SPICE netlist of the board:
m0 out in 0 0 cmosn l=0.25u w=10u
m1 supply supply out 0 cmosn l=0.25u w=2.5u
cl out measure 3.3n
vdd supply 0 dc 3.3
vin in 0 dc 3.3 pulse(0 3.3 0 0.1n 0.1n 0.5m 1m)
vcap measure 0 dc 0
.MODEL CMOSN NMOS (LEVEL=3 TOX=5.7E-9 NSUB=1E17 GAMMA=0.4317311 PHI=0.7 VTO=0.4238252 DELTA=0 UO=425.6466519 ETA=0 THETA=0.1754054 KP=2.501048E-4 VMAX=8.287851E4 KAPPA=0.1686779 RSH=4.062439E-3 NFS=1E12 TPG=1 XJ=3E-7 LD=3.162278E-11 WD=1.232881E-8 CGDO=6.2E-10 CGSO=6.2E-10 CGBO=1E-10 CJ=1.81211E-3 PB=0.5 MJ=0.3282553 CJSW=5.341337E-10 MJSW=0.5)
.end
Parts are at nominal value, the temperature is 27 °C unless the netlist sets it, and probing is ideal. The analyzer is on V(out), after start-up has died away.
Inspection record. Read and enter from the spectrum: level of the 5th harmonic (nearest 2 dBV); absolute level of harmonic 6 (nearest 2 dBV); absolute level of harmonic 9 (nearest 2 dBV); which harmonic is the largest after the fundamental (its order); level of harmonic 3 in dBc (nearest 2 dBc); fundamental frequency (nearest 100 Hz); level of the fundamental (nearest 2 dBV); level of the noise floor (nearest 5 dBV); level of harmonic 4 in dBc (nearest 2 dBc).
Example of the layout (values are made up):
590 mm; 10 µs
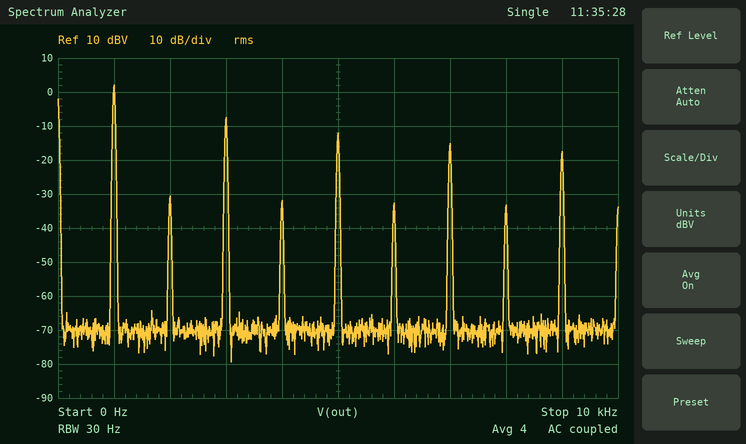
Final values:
-12 dBV; -32 dBV; -18 dBV; 3; -10 dBc; 1.0 kHz; 2 dBV; -70 dBV; -34 dBc
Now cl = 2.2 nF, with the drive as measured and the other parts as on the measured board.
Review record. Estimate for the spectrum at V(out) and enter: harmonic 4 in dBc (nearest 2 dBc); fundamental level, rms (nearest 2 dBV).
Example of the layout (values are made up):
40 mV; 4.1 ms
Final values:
-36 dBc; 2 dBV
